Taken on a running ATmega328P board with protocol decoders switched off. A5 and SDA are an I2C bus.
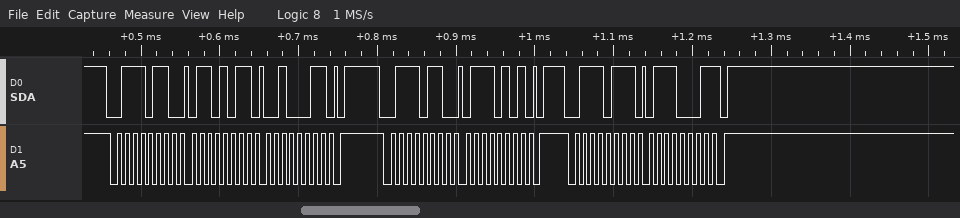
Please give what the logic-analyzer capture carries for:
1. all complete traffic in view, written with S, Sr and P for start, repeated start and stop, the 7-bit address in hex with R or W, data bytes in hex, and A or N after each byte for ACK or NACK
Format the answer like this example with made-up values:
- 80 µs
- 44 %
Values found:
- S 3BW A 6B A 23 A P S 3BW A 75 A P S 3BR A 71 N P
